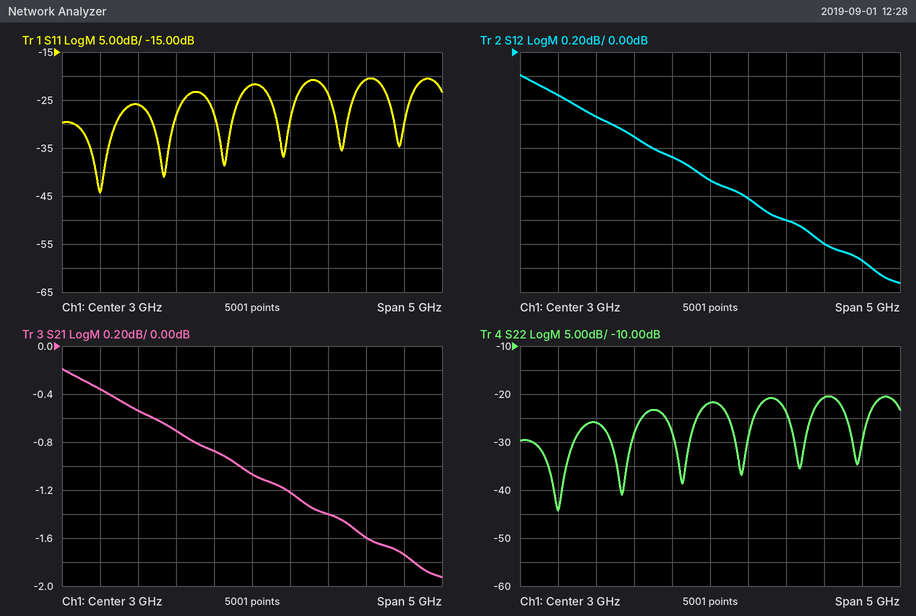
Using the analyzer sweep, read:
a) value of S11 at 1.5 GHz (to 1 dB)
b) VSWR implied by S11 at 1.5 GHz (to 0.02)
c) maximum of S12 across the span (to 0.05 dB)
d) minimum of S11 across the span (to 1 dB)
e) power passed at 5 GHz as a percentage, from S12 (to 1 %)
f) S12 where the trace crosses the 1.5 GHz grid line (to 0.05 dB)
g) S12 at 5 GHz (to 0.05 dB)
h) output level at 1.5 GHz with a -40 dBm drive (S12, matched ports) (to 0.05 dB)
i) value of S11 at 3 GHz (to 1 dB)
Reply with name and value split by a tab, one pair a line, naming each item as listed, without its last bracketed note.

value of S11 at 1.5 GHz	-26 dB
VSWR implied by S11 at 1.5 GHz	1.10
maximum of S12 across the span	-0.20 dB
minimum of S11 across the span	-44 dB
power passed at 5 GHz as a percentage, from S12	67 %
S12 where the trace crosses the 1.5 GHz grid line	-0.55 dB
S12 at 5 GHz	-1.75 dB
output level at 1.5 GHz with a -40 dBm drive (S12, matched ports)	-40.55 dBm
value of S11 at 3 GHz	-22 dB
